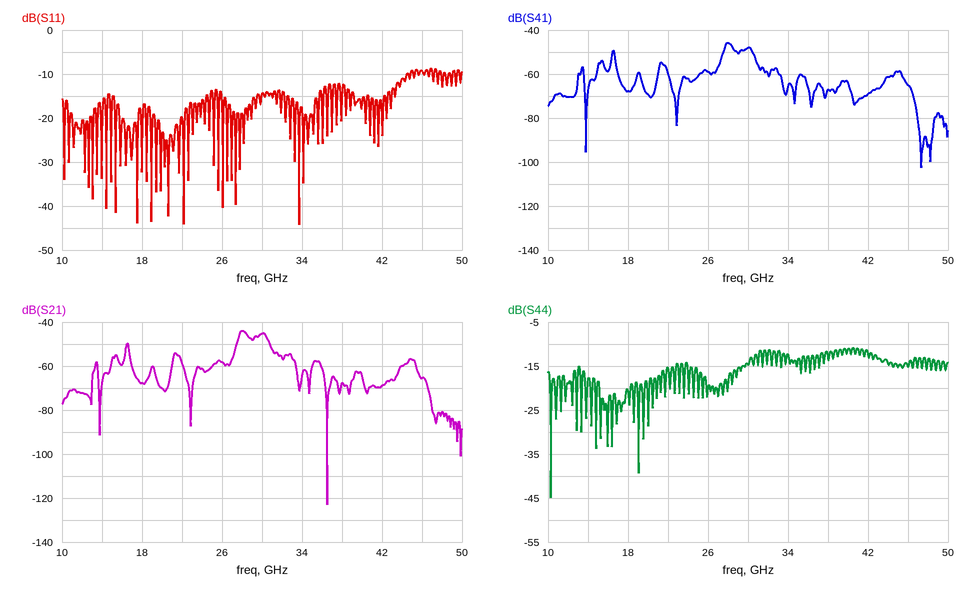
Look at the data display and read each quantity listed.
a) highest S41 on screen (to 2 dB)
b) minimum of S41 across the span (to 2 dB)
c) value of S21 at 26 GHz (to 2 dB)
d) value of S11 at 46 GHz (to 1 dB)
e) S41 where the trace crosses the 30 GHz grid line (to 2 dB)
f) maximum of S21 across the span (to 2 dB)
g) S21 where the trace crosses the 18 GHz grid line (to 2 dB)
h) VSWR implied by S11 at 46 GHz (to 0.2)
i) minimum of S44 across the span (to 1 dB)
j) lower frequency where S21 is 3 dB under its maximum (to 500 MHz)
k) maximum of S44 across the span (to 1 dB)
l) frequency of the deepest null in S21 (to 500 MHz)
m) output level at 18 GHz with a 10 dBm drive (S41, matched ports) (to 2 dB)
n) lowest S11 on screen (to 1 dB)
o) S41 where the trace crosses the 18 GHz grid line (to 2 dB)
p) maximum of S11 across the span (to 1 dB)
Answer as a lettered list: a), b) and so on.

a) -46 dB
b) -102 dB
c) -58 dB
d) -9 dB
e) -48 dB
f) -44 dB
g) -68 dB
h) 2.0
i) -45 dB
j) 27.5 GHz
k) -11 dB
l) 36.5 GHz
m) -58 dBm
n) -44 dB
o) -68 dB
p) -9 dB
